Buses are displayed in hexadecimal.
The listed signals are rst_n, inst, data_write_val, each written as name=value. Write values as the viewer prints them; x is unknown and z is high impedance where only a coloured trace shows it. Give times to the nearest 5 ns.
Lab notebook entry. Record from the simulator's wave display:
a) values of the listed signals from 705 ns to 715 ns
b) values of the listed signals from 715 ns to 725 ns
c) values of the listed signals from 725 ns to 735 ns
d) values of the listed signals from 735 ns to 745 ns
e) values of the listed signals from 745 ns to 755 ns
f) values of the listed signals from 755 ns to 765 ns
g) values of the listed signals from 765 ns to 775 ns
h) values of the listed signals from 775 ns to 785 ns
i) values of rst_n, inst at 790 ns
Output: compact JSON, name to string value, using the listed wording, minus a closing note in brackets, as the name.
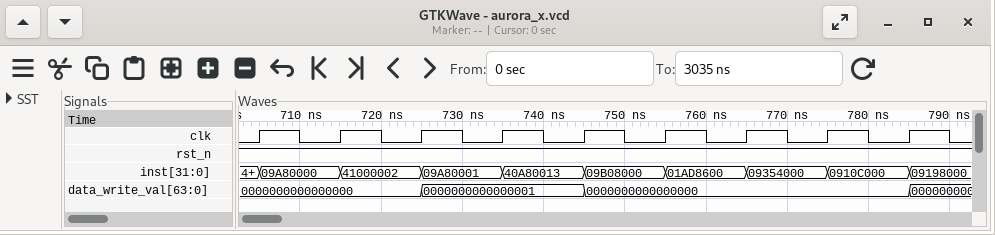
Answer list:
{"values of the listed signals from 705 ns to 715 ns": "rst_n=1, inst=09A80000, data_write_val=0000000000000000", "values of the listed signals from 715 ns to 725 ns": "rst_n=1, inst=41000002, data_write_val=0000000000000000", "values of the listed signals from 725 ns to 735 ns": "rst_n=1, inst=09A80001, data_write_val=0000000000000001", "values of the listed signals from 735 ns to 745 ns": "rst_n=1, inst=40A80013, data_write_val=0000000000000001", "values of the listed signals from 745 ns to 755 ns": "rst_n=1, inst=09B08000, data_write_val=0000000000000000", "values of the listed signals from 755 ns to 765 ns": "rst_n=1, inst=01AD8600, data_write_val=0000000000000000", "values of the listed signals from 765 ns to 775 ns": "rst_n=1, inst=09354000, data_write_val=0000000000000000", "values of the listed signals from 775 ns to 785 ns": "rst_n=1, inst=0910C000, data_write_val=0000000000000000", "values of rst_n, inst at 790 ns": "rst_n=1, inst=09198000"}
